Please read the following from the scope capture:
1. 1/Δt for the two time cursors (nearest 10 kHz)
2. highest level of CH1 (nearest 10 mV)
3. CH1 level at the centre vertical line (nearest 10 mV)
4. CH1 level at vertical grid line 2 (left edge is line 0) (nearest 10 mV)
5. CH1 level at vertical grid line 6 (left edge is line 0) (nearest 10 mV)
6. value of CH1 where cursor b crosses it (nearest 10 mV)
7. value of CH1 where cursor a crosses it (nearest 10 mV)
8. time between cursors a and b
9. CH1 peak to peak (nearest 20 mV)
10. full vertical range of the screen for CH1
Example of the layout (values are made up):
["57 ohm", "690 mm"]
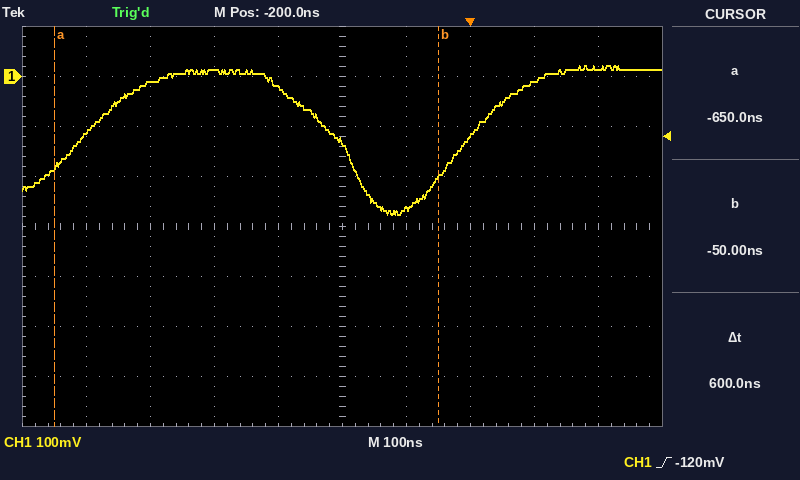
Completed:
["1.67 MHz", "20 mV", "-130 mV", "-10 mV", "-260 mV", "-200 mV", "-180 mV", "600 ns", "300 mV", "800 mV"]
